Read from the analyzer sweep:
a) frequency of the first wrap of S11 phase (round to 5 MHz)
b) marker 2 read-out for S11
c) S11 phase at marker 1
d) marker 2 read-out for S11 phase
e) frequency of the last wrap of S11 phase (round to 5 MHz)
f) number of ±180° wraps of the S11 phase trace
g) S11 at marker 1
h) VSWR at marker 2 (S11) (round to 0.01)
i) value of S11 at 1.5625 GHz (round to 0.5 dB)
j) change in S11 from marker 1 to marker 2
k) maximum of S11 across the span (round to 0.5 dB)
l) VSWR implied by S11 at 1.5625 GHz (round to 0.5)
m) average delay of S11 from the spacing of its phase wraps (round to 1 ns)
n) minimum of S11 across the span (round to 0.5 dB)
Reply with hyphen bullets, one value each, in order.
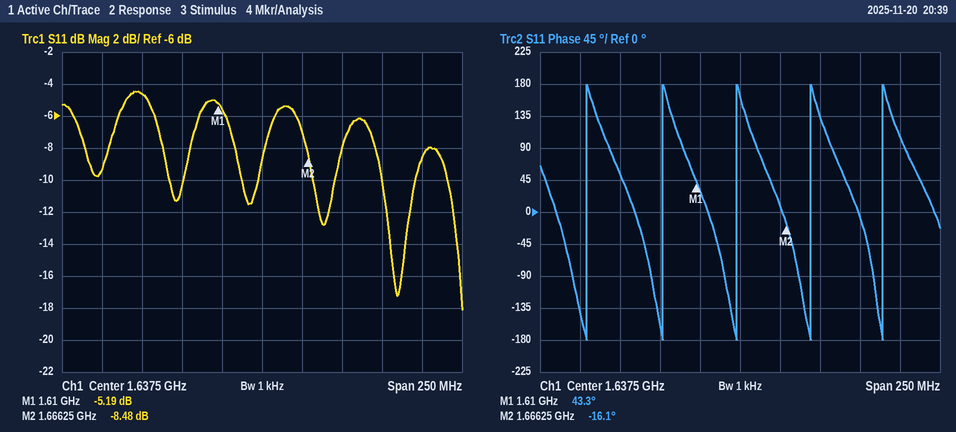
- 1.540 GHz
- -8.48 dB
- 43.3°
- -16.1°
- 1.725 GHz
- 5
- -5.19 dB
- 2.21
- -4.5 dB
- -3.29 dB
- -4.5 dB
- 4.0
- 22 ns
- -18.0 dB
